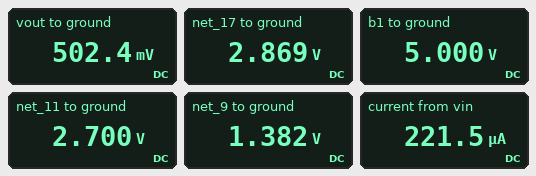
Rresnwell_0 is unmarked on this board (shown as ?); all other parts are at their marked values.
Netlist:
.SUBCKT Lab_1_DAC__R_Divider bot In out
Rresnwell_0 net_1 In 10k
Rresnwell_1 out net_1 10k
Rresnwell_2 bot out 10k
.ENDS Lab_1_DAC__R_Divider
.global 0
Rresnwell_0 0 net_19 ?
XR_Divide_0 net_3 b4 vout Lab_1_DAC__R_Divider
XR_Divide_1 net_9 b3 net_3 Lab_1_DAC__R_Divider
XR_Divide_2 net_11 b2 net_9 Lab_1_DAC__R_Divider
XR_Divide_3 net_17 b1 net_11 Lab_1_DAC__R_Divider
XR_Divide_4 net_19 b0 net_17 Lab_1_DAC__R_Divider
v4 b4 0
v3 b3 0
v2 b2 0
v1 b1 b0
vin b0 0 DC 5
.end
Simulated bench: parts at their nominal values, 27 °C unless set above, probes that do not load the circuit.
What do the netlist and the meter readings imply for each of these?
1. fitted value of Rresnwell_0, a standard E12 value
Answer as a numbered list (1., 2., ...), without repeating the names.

1. 22 kΩ
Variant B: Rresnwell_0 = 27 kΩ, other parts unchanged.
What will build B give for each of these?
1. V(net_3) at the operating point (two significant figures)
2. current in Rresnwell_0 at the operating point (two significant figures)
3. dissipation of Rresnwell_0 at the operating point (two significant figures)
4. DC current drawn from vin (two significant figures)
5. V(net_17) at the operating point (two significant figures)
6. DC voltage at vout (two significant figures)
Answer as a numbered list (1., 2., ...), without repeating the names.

1. 770 mV
2. 80 µA
3. 170 µW
4. 210 µA
5. 3.0 V
6. 510 mV
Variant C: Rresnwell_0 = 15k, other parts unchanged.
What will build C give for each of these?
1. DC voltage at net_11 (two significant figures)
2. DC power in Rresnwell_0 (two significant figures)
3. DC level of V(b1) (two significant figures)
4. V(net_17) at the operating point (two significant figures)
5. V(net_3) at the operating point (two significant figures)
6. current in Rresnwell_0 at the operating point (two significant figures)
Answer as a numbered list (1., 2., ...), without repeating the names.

1. 2.6 V
2. 170 µW
3. 5.0 V
4. 2.7 V
5. 730 mV
6. 110 µA
